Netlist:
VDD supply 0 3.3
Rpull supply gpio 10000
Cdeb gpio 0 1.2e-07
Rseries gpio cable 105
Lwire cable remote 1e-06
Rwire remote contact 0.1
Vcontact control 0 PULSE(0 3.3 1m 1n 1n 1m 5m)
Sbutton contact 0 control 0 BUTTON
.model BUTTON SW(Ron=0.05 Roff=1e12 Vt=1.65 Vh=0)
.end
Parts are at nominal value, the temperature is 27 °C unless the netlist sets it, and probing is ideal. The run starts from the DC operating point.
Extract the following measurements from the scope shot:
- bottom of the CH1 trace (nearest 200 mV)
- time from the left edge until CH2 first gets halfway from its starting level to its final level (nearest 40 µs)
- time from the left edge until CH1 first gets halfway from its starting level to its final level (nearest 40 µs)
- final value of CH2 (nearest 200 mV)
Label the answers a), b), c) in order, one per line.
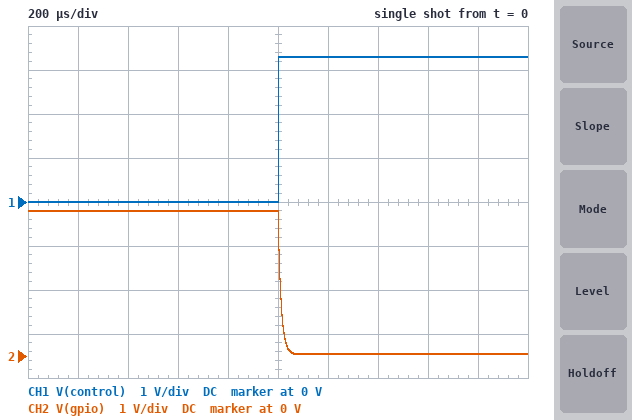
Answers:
a) 0 V
b) 1.00 ms
c) 1.00 ms
d) 0 V
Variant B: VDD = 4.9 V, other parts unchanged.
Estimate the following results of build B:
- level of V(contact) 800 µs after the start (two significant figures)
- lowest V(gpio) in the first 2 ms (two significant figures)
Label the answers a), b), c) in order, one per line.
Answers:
a) 4.9 V
b) 51 mV
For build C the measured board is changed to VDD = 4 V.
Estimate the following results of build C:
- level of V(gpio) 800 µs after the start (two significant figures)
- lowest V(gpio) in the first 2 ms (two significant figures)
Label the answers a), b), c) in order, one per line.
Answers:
a) 4.0 V
b) 42 mV
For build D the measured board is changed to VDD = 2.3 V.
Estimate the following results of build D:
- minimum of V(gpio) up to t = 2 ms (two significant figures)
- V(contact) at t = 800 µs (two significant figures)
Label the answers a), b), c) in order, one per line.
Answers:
a) 24 mV
b) 2.3 V
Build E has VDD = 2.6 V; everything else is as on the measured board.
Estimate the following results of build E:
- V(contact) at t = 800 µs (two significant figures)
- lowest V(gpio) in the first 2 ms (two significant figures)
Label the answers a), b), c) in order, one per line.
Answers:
a) 2.6 V
b) 27 mV
